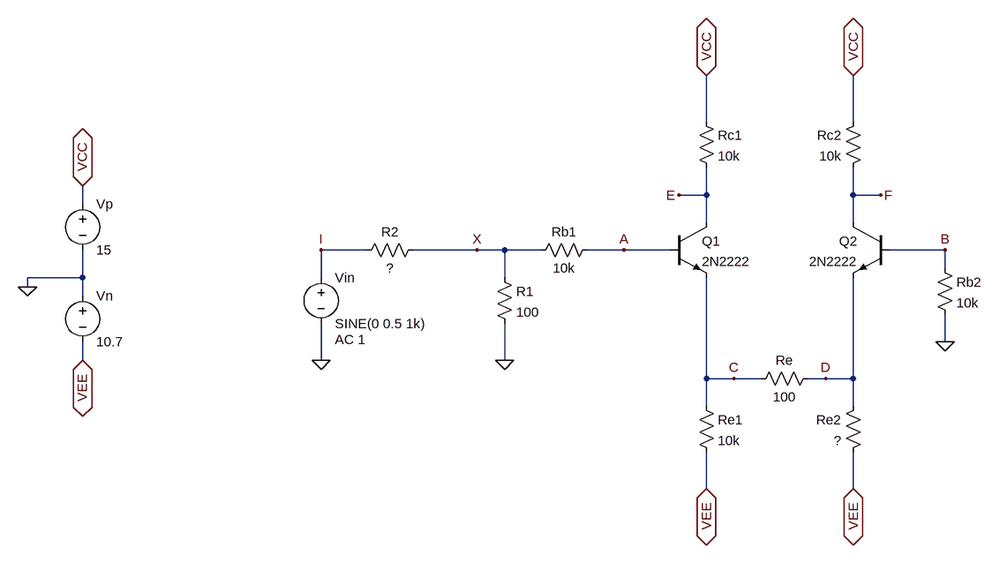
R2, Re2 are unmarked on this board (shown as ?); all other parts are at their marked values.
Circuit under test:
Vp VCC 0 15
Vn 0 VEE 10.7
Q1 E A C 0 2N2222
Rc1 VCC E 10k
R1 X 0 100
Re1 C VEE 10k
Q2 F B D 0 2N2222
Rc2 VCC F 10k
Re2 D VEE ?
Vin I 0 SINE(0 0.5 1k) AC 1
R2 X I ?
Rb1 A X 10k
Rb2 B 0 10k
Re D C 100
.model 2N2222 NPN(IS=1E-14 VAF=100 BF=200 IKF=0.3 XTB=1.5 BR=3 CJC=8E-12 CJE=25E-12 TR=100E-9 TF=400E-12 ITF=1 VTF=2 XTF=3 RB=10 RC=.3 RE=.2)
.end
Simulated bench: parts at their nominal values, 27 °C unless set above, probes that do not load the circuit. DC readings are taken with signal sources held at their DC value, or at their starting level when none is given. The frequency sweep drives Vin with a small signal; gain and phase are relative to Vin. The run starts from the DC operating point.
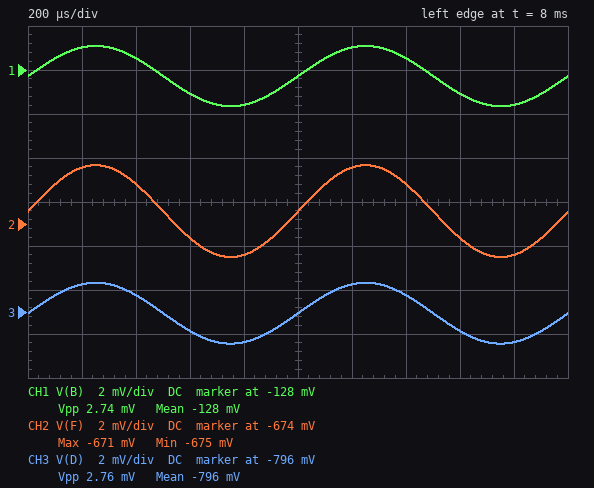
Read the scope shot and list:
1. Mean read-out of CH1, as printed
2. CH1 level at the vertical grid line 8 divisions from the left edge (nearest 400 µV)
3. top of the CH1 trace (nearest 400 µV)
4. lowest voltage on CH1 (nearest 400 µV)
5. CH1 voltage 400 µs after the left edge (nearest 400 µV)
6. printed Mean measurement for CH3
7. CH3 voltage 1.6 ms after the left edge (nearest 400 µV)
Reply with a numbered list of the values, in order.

1. -128 mV
2. -129.2 mV
3. -126.8 mV
4. -129.6 mV
5. -127.6 mV
6. -796 mV
7. -796.8 mV
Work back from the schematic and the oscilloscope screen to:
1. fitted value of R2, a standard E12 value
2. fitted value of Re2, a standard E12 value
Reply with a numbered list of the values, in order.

1. 33 kΩ
2. 4.7 kΩ
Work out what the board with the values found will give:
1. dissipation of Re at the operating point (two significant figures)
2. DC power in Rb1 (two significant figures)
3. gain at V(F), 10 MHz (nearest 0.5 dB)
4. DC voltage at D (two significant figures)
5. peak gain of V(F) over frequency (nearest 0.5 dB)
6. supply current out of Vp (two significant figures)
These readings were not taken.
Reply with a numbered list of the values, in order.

1. 28 µW
2. 580 nW
3. -67.5 dB
4. -800 mV
5. -47.5 dB
6. 3.1 mA
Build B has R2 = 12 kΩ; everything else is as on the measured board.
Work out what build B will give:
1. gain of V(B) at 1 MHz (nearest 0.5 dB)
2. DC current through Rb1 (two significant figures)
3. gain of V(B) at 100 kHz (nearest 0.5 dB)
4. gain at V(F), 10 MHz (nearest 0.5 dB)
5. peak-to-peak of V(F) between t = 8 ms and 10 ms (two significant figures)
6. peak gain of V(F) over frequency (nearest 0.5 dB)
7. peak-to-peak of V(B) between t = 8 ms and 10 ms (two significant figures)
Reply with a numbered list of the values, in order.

1. -53.0 dB
2. 7.6 µA
3. -43.0 dB
4. -59.0 dB
5. 11 mV
6. -39.0 dB
7. 7.5 mV
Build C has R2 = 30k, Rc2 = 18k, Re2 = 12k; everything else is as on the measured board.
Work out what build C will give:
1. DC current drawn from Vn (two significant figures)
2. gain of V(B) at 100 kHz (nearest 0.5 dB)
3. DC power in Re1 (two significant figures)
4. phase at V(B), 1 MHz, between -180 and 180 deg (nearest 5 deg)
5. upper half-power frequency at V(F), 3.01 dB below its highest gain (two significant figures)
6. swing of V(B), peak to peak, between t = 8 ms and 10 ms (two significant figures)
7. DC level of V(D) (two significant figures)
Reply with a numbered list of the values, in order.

1. 1.8 mA
2. -51.5 dB
3. 10 mW
4. -35 deg
5. 69 kHz
6. 2.5 mV
7. -700 mV
